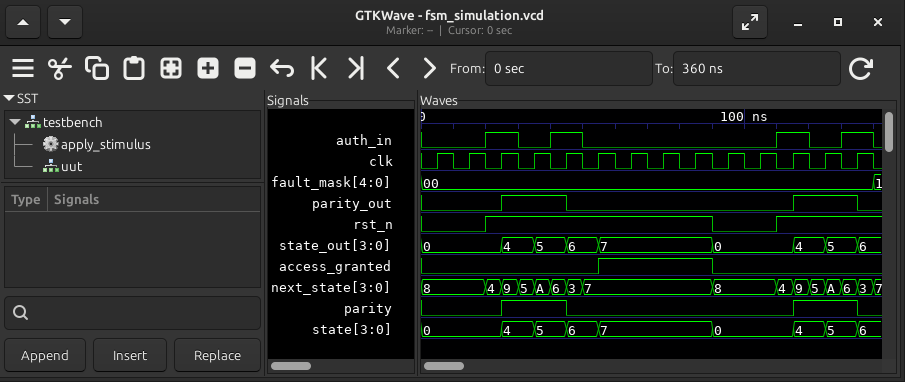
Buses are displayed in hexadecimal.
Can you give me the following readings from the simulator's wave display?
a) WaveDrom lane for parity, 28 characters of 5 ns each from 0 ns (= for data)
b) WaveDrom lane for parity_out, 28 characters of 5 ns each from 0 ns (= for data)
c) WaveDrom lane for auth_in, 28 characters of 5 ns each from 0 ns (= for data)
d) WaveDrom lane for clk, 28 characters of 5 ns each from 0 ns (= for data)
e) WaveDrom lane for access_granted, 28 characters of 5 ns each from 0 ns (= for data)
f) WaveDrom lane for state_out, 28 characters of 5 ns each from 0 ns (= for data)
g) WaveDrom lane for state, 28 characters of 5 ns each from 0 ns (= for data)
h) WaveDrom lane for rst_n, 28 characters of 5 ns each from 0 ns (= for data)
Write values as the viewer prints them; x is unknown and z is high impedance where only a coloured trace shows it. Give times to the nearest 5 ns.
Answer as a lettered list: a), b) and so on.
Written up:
a) {name: 'parity', wave: '0....1...0.............1...0'}
b) {name: 'parity_out', wave: '0....1...0.............1...0'}
c) {name: 'auth_in', wave: '0...1.0.1.0...........1.0.1.'}
d) {name: 'clk', wave: '0101010101010101010101010101'}
e) {name: 'access_granted', wave: '0..........1......0.........'}
f) {name: 'state_out', wave: '=....=.=.=.=......=....=.=.=', data: '0 4 5 6 7 0 4 5 6'}
g) {name: 'state', wave: '=....=.=.=.=......=....=.=.=', data: '0 4 5 6 7 0 4 5 6'}
h) {name: 'rst_n', wave: '0...1.............0...1.....'}
